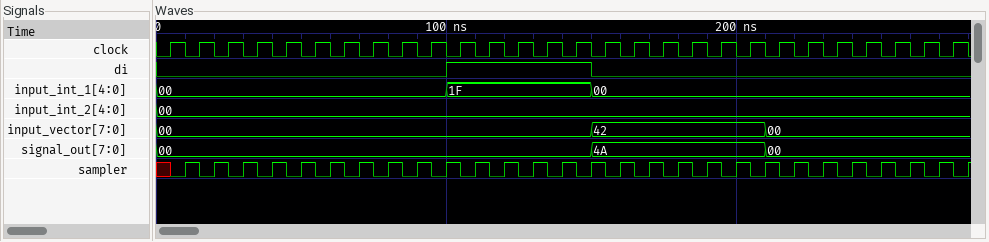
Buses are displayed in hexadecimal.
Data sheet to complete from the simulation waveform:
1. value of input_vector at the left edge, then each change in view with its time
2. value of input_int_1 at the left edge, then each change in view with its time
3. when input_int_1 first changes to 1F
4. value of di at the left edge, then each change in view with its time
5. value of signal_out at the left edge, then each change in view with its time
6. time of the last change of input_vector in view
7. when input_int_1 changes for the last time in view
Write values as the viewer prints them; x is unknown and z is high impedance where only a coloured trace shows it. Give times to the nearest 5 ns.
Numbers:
00, 42 at 150 ns, 00 at 210 ns
00, 1F at 100 ns, 00 at 150 ns
100 ns
0, 1 at 100 ns, 0 at 150 ns
00, 4A at 150 ns, 00 at 210 ns
210 ns
150 ns
